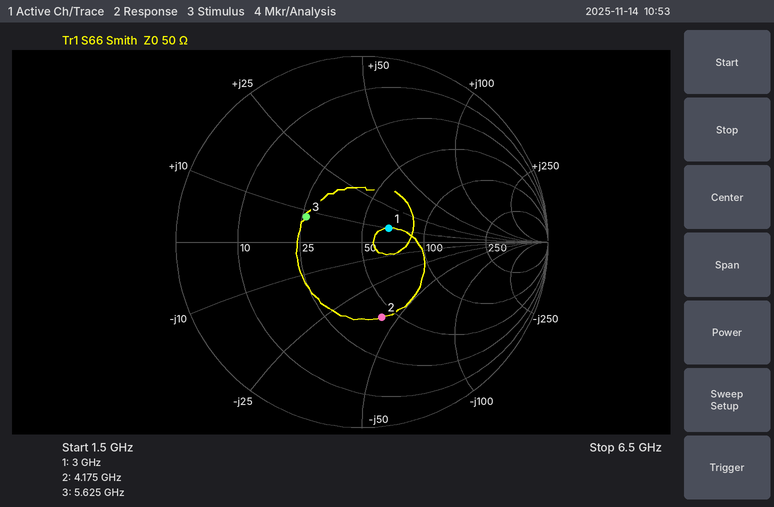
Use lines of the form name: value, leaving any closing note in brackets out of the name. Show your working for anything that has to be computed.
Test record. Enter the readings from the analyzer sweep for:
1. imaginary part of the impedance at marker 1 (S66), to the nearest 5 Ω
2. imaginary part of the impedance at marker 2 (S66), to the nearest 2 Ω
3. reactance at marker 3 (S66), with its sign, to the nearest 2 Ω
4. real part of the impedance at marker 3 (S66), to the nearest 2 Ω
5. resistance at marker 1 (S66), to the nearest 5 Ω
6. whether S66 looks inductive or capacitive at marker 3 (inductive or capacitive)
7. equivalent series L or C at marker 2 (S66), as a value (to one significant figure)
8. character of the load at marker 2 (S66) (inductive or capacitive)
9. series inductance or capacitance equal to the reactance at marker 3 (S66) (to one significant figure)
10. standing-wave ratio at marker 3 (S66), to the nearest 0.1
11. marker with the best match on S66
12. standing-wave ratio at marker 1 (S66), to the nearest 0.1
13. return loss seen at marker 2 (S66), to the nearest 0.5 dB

imaginary part of the impedance at marker 1 (S66), to the nearest 5 Ω: +10 Ω
imaginary part of the impedance at marker 2 (S66), to the nearest 2 Ω: -42 Ω
reactance at marker 3 (S66), with its sign, to the nearest 2 Ω: +8 Ω
real part of the impedance at marker 3 (S66), to the nearest 2 Ω: 26 Ω
resistance at marker 1 (S66), to the nearest 5 Ω: 65 Ω
whether S66 looks inductive or capacitive at marker 3: inductive
equivalent series L or C at marker 2 (S66), as a value: C = 1/(2π × 4.175 GHz × 42 Ω) ≈ 908 fF, so 900 fF to one significant figure
character of the load at marker 2 (S66): capacitive
series inductance or capacitance equal to the reactance at marker 3 (S66): L = 8 Ω/(2π × 5.625 GHz) ≈ 226 pH, so 200 pH to one significant figure
standing-wave ratio at marker 3 (S66), to the nearest 0.1: 2.0
marker with the best match on S66: marker 1
standing-wave ratio at marker 1 (S66), to the nearest 0.1: 1.4
return loss seen at marker 2 (S66), to the nearest 0.5 dB: 7.5 dB
